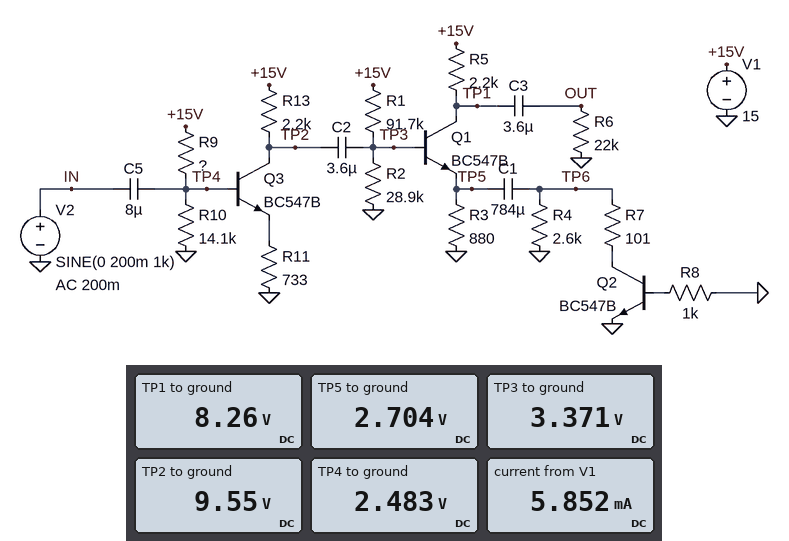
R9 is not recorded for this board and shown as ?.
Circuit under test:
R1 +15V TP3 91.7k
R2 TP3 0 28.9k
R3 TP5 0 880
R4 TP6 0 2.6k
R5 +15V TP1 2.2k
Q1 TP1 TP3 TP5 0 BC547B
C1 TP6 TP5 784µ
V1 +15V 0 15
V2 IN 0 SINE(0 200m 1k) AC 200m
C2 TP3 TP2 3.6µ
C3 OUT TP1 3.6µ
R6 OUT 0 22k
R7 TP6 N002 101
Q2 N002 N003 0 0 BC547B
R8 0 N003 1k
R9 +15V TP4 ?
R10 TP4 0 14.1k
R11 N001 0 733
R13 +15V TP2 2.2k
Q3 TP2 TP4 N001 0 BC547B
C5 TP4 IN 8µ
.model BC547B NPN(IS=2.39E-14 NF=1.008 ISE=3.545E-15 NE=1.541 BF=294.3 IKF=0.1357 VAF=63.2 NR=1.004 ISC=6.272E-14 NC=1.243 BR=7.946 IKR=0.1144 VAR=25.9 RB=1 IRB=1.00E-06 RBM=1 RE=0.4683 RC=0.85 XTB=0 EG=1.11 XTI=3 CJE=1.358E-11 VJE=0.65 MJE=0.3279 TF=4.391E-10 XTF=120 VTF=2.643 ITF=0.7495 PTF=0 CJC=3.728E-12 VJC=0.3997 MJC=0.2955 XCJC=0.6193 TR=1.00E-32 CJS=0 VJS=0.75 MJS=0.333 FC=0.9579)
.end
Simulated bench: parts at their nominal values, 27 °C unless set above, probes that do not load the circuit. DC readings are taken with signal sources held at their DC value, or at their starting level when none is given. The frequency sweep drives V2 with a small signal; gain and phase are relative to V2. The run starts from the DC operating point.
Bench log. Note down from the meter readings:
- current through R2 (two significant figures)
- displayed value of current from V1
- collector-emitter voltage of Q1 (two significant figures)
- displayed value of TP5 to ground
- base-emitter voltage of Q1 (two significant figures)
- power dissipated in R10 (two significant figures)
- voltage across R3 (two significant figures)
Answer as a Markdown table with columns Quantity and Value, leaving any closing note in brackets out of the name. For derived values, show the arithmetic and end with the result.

| Quantity | Value |
|---|---|
| current through R2 | (3.371 V) / 28.9 kΩ = 120 µA |
| displayed value of current from V1 | 5.852 mA |
| collector-emitter voltage of Q1 | 8.26 V - 2.704 V = 5.6 V |
| displayed value of TP5 to ground | 2.704 V |
| base-emitter voltage of Q1 | 3.371 V - 2.704 V = 670 mV |
| power dissipated in R10 | (2.483 V)^2 / 14.1 kΩ = 440 µW |
| voltage across R3 | 2.704 V = 2.7 V |
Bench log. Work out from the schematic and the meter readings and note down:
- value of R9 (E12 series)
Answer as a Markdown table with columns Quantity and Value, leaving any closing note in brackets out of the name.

| Quantity | Value |
|---|---|
| value of R9 | 68 kΩ |
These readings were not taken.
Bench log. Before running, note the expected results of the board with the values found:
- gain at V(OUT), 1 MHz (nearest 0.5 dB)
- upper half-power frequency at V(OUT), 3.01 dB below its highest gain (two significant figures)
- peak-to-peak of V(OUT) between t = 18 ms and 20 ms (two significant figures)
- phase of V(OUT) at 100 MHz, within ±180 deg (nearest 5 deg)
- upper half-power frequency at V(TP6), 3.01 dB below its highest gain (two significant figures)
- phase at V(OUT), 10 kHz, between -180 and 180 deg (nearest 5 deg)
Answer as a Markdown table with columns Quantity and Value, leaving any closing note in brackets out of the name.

| Quantity | Value |
|---|---|
| gain at V(OUT), 1 MHz | 18.0 dB |
| upper half-power frequency at V(OUT), 3.01 dB below its highest gain | 7.5 MHz |
| peak-to-peak of V(OUT) between t = 18 ms and 20 ms | 3.2 V |
| phase of V(OUT) at 100 MHz, within ±180 deg | 160 deg |
| upper half-power frequency at V(TP6), 3.01 dB below its highest gain | 7.5 MHz |
| phase at V(OUT), 10 kHz, between -180 and 180 deg | 0 deg |
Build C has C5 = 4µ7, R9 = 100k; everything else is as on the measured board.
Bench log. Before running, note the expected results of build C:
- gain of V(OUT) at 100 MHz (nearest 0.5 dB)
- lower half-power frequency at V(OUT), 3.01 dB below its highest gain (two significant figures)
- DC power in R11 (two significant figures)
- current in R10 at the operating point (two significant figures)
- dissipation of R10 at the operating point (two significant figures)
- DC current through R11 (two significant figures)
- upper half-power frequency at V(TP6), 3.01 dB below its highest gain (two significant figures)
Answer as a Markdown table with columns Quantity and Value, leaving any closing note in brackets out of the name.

| Quantity | Value |
|---|---|
| gain of V(OUT) at 100 MHz | -2.5 dB |
| lower half-power frequency at V(OUT), 3.01 dB below its highest gain | 4.5 Hz |
| DC power in R11 | 1.8 mW |
| current in R10 at the operating point | 130 µA |
| dissipation of R10 at the operating point | 230 µW |
| DC current through R11 | 1.6 mA |
| upper half-power frequency at V(TP6), 3.01 dB below its highest gain | 7.6 MHz |
